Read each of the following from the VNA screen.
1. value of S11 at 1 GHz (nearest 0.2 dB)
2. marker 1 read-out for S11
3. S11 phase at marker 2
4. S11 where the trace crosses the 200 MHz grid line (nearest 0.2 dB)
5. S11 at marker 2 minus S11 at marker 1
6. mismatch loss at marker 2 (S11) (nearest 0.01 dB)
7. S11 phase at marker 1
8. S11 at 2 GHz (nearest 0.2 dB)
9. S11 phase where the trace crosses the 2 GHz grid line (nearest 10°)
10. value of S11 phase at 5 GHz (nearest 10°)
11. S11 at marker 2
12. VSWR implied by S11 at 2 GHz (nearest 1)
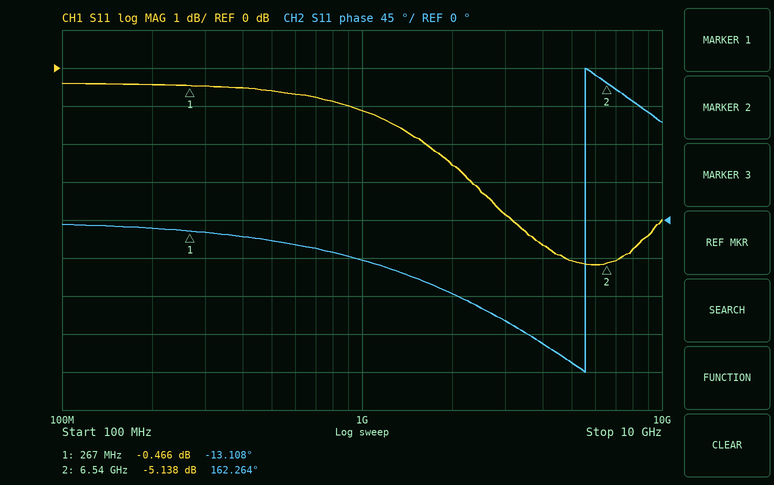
-1.2 dB
-0.466 dB
162.264°
-0.4 dB
-4.672 dB
1.59 dB
-13.108°
-2.6 dB
-90°
-170°
-5.138 dB
7
